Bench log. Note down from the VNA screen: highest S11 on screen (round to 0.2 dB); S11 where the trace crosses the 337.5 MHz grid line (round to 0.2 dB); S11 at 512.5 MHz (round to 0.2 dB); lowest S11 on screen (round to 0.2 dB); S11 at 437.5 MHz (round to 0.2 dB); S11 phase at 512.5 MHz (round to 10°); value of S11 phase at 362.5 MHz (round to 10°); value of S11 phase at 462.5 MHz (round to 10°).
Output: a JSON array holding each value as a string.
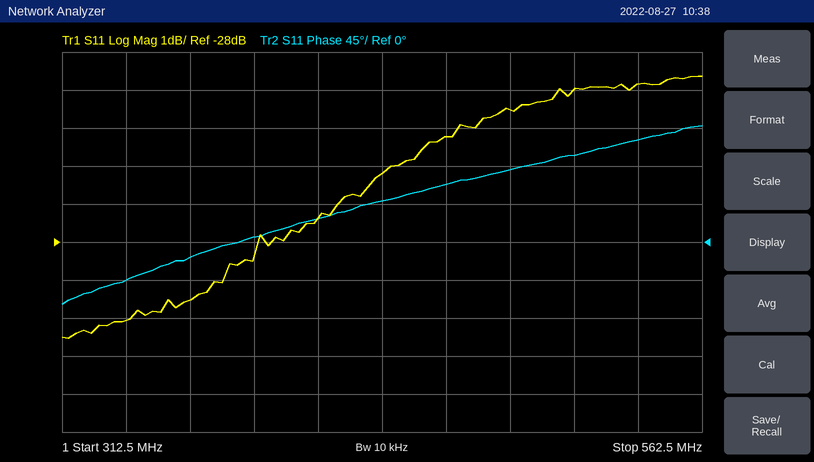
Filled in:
["-23.6 dB", "-30.0 dB", "-24.0 dB", "-30.6 dB", "-26.2 dB", "100°", "-20°", "70°"]
